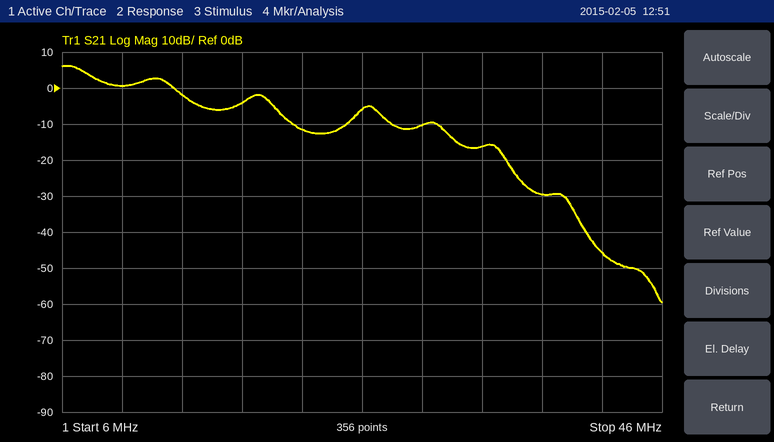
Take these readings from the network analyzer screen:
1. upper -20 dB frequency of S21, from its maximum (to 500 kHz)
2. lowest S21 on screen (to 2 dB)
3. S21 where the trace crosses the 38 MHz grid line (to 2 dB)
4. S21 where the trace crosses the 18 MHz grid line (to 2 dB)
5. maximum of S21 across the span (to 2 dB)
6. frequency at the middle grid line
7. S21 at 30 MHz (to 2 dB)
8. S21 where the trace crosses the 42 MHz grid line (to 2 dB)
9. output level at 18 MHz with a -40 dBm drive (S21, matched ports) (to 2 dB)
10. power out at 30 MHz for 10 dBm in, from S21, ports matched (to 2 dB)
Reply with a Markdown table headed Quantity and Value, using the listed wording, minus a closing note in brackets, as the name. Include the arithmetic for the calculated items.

| Quantity | Value |
|---|---|
| upper -20 dB frequency of S21, from its maximum | 32.0 MHz |
| lowest S21 on screen | -60 dB |
| S21 where the trace crosses the 38 MHz grid line | -30 dB |
| S21 where the trace crosses the 18 MHz grid line | -4 dB |
| maximum of S21 across the span | 6 dB |
| frequency at the middle grid line | 26 MHz |
| S21 at 30 MHz | -10 dB |
| S21 where the trace crosses the 42 MHz grid line | -46 dB |
| output level at 18 MHz with a -40 dBm drive (S21, matched ports) | -40 dBm + (-4 dB) = -44 dBm |
| power out at 30 MHz for 10 dBm in, from S21, ports matched | 10 dBm + (-10 dB) = 0 dBm |
